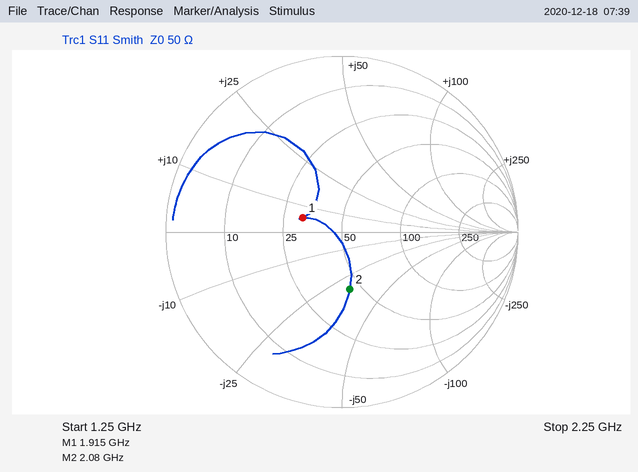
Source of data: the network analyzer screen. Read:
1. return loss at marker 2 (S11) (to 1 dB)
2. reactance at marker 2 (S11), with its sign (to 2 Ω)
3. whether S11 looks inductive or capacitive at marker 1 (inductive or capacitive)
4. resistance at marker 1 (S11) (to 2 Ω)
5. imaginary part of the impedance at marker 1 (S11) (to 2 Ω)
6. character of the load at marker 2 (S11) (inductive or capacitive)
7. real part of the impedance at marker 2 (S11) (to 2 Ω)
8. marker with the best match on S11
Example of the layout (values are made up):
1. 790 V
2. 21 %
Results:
1. 10 dB
2. -32 Ω
3. inductive
4. 32 Ω
5. +6 Ω
6. capacitive
7. 44 Ω
8. marker 1
